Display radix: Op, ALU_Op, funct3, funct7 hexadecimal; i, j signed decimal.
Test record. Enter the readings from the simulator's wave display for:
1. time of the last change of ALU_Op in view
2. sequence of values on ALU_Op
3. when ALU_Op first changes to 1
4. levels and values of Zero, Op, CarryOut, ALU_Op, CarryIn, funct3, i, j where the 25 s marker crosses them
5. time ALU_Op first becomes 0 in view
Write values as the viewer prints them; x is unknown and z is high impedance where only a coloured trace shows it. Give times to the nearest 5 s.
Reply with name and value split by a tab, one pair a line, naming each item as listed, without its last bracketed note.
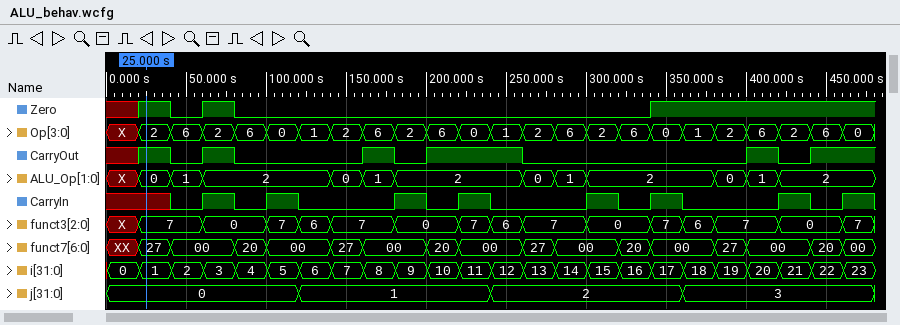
time of the last change of ALU_Op in view	420 s
sequence of values on ALU_Op	X, 0, 1, 2, 0, 1, 2, 0, 1, 2, 0, 1, 2
when ALU_Op first changes to 1	40 s
levels and values of Zero, Op, CarryOut, ALU_Op, CarryIn, funct3, i, j where the 25 s marker crosses them	Zero=1, Op=2, CarryOut=1, ALU_Op=0, CarryIn=x, funct3=7, i=1, j=0
time ALU_Op first becomes 0 in view	20 s
